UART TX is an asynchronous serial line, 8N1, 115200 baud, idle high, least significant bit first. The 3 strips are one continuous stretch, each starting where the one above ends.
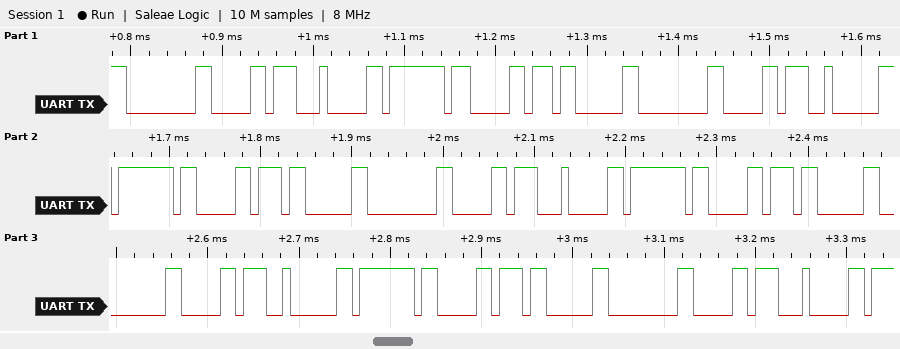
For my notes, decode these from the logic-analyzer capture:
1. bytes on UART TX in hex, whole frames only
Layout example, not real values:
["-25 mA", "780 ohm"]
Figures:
["0x00 0xB0 0x04 0x7F 0xB0 0x03 0x00 0xB0 0x02 0x7F 0xB0 0x03 0x00 0xB0 0x04 0x7F 0xB0 0x03 0x00 0xB0 0x02 0x7F 0xB0 0x03 0x00 0xB0 0x04"]
